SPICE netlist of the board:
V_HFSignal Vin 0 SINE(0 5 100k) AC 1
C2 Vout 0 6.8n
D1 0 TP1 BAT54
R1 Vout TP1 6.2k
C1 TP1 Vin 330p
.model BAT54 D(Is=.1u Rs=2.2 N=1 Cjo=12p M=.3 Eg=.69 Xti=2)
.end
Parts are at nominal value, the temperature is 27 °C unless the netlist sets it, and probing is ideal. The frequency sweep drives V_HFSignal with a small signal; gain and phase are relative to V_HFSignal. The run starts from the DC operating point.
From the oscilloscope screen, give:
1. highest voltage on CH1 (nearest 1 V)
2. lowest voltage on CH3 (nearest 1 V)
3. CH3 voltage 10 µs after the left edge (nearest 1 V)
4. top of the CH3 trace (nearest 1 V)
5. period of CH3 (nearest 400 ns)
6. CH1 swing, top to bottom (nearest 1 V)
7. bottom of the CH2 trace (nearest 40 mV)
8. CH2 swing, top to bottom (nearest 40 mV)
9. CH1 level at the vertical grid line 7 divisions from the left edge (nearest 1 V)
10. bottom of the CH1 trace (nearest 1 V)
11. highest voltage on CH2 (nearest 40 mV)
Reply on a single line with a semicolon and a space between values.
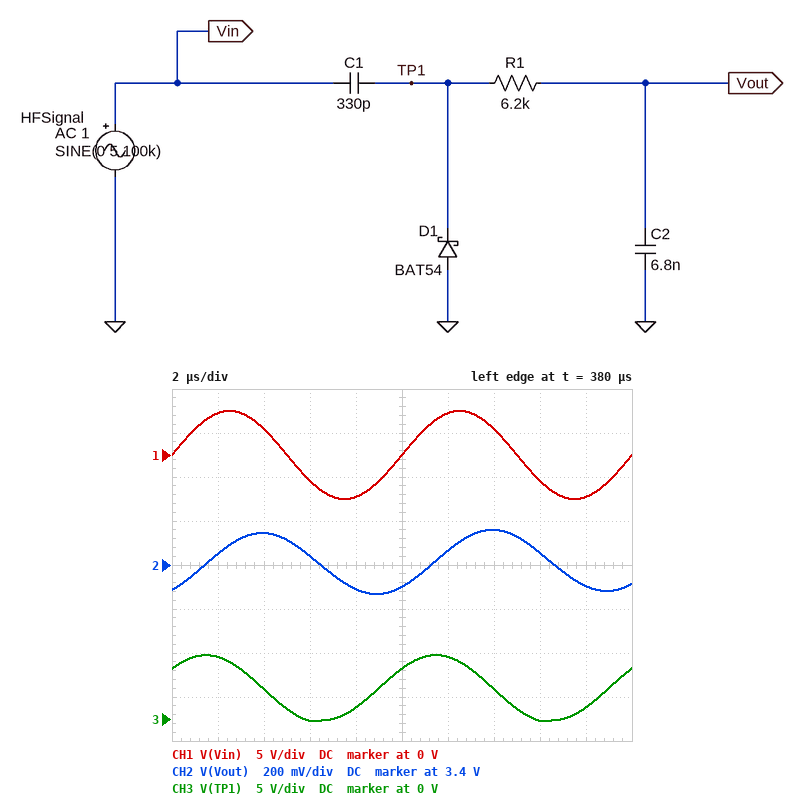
5 V; 0 V; 6 V; 7 V; 10.0 µs; 10 V; 3.28 V; 280 mV; 3 V; -5 V; 3.56 V
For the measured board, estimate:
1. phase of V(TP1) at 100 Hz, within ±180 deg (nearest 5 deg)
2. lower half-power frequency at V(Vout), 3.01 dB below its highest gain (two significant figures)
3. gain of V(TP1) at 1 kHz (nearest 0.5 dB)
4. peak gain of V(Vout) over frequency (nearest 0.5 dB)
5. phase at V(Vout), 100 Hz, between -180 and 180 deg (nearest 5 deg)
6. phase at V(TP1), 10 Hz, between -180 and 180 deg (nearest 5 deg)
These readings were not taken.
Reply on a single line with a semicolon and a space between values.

40 deg; 84 Hz; -26.5 dB; -27.0 dB; 40 deg; 85 deg
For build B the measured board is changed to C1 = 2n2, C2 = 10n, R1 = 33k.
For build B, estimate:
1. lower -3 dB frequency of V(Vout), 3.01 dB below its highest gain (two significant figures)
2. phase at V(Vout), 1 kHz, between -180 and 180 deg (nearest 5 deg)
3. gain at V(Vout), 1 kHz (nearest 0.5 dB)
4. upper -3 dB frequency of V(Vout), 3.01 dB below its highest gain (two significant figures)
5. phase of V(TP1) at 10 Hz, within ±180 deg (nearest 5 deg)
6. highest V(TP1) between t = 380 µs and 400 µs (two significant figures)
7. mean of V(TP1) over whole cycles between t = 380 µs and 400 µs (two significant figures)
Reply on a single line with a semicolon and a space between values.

45 Hz; -15 deg; -16.0 dB; 3.0 kHz; 80 deg; 9.7 V; 4.7 V
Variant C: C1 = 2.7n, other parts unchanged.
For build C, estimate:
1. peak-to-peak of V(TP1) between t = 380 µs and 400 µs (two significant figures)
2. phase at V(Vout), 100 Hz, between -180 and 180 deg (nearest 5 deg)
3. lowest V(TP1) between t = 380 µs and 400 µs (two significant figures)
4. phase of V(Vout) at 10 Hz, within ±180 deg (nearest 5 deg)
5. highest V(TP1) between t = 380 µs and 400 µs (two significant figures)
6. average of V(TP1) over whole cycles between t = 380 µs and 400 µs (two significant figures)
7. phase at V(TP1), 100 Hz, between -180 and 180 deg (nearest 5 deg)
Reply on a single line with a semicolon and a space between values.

9.9 V; 30 deg; -170 mV; 80 deg; 9.7 V; 4.8 V; 35 deg
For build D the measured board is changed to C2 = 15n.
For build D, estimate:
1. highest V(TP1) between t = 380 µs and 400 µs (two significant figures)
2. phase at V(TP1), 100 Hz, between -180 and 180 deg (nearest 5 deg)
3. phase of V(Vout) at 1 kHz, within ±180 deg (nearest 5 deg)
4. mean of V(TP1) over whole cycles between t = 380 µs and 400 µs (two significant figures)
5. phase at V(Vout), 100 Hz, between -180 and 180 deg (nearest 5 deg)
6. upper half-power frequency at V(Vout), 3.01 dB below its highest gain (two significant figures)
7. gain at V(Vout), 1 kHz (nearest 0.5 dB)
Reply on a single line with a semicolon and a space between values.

6.7 V; 25 deg; 0 deg; 3.0 V; 20 deg; 79 kHz; -33.5 dB
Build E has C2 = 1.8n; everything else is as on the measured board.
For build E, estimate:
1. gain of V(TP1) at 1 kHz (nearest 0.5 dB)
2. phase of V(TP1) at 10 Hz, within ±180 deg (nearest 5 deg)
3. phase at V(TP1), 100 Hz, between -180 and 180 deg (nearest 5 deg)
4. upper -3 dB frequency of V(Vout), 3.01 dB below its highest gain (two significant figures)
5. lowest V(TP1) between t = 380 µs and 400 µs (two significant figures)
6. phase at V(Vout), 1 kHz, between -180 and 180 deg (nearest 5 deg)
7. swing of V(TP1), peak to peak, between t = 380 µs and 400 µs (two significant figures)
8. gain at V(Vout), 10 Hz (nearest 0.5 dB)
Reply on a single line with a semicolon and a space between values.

-16.5 dB; 90 deg; 70 deg; 91 kHz; -120 mV; 15 deg; 7.3 V; -45.5 dB
